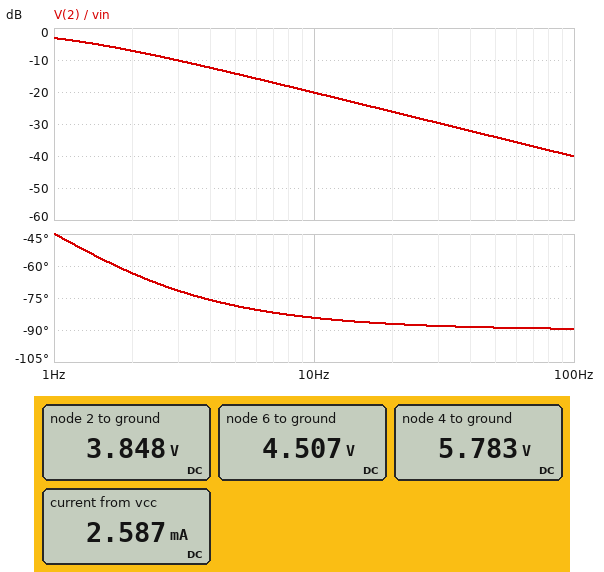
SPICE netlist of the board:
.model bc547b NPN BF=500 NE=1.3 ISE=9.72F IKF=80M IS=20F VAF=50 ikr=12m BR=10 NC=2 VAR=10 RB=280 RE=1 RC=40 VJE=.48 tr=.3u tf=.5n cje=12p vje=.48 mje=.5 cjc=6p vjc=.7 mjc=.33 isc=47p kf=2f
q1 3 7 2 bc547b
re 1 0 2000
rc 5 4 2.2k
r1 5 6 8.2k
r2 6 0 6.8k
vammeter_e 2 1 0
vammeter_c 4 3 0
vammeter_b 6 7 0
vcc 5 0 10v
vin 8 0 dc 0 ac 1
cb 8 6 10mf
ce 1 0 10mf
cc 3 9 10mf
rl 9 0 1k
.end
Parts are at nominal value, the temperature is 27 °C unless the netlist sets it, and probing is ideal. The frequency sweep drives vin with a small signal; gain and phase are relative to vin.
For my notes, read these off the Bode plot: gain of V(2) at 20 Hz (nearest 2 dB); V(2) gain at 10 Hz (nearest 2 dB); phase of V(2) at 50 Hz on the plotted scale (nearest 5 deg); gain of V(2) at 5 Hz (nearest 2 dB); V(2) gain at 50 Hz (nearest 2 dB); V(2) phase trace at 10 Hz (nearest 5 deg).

-26 dB
-20 dB
-90 deg
-14 dB
-34 dB
-85 deg
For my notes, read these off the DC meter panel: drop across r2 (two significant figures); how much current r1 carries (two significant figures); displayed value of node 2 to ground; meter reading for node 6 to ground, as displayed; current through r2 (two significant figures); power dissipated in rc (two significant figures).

4.5 V
670 µA
3.848 V
4.507 V
660 µA
8.1 mW
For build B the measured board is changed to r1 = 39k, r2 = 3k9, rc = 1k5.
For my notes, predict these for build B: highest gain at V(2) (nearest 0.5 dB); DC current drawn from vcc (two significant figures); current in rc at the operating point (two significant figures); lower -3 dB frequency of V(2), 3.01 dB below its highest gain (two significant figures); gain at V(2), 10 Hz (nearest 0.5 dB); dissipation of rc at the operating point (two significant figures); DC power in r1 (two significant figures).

-1.0 dB
390 µA
160 µA
4.2 mHz
-40.5 dB
38 µW
2.1 mW
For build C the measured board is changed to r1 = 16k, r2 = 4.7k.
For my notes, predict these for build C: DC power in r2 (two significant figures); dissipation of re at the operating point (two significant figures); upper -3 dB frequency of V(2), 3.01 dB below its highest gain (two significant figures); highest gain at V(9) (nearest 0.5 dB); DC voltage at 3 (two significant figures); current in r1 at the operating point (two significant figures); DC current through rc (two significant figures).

1.1 mW
1.3 mW
480 mHz
26.0 dB
8.2 V
480 µA
810 µA
